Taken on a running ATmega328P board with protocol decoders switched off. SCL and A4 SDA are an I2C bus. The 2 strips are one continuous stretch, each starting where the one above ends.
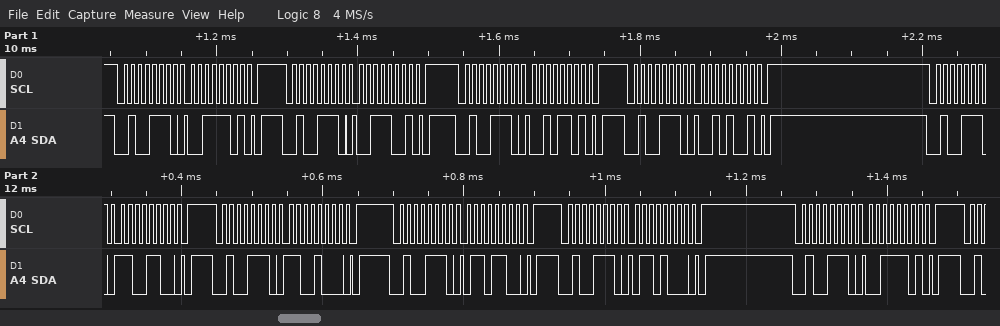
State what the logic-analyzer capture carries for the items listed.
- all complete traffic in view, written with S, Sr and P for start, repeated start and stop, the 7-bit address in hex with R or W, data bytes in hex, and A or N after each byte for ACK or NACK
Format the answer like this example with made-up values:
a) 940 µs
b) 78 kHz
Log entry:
a) S 27W A 3D A P S 27W A 39 A P S 27W A 2D A P S 27W A 29 A P S 27W A CC A P S 27W A C8 A P S 27W A 6C A P S 27W A 68 A P S 27W A 3D A P
